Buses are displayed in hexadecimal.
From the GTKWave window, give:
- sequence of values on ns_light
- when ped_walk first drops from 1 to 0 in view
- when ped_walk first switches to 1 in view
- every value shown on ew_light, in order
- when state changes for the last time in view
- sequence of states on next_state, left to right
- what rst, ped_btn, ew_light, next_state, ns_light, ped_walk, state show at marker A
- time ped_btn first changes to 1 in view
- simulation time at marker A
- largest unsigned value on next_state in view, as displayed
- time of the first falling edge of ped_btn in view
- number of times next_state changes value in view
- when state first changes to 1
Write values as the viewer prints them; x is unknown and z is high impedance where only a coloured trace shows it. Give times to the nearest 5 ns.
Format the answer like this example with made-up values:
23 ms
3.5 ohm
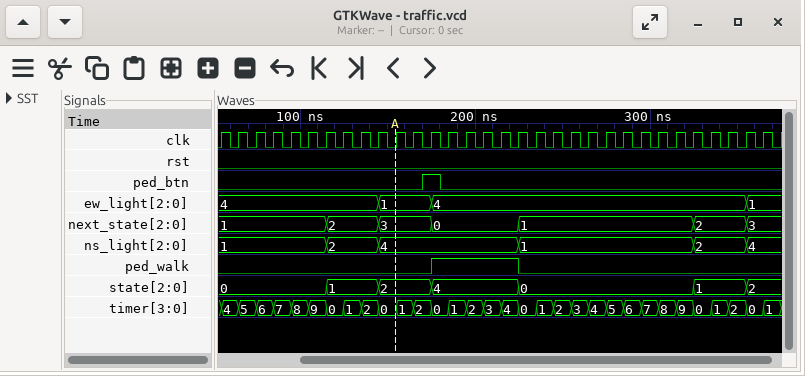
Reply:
1, 2, 4, 1, 2, 4
225 ns
175 ns
4, 1, 4, 1
355 ns
1, 2, 3, 0, 1, 2, 3
rst=0, ped_btn=0, ew_light=1, next_state=3, ns_light=4, ped_walk=0, state=2
170 ns
155 ns
3
180 ns
6
115 ns
